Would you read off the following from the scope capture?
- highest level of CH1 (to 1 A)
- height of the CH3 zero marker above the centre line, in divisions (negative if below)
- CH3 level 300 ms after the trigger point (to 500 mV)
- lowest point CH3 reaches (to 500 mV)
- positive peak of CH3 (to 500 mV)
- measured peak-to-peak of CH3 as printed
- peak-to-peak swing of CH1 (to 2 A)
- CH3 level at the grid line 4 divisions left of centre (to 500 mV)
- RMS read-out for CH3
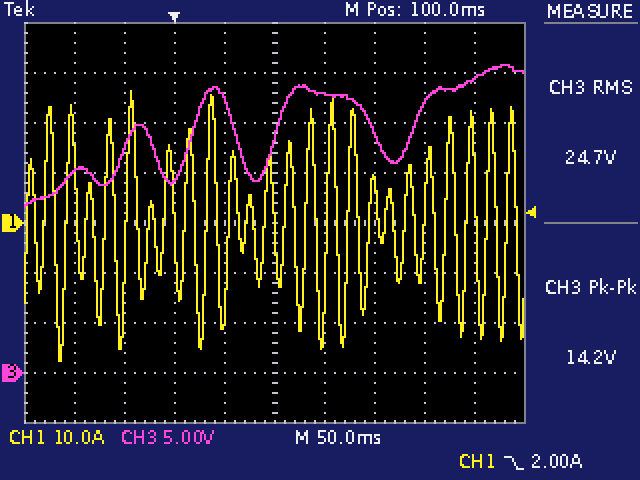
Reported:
26 A
-3.0 div
29.5 V
16.5 V
31.0 V
14.2 V
54 A
20.0 V
24.7 V
